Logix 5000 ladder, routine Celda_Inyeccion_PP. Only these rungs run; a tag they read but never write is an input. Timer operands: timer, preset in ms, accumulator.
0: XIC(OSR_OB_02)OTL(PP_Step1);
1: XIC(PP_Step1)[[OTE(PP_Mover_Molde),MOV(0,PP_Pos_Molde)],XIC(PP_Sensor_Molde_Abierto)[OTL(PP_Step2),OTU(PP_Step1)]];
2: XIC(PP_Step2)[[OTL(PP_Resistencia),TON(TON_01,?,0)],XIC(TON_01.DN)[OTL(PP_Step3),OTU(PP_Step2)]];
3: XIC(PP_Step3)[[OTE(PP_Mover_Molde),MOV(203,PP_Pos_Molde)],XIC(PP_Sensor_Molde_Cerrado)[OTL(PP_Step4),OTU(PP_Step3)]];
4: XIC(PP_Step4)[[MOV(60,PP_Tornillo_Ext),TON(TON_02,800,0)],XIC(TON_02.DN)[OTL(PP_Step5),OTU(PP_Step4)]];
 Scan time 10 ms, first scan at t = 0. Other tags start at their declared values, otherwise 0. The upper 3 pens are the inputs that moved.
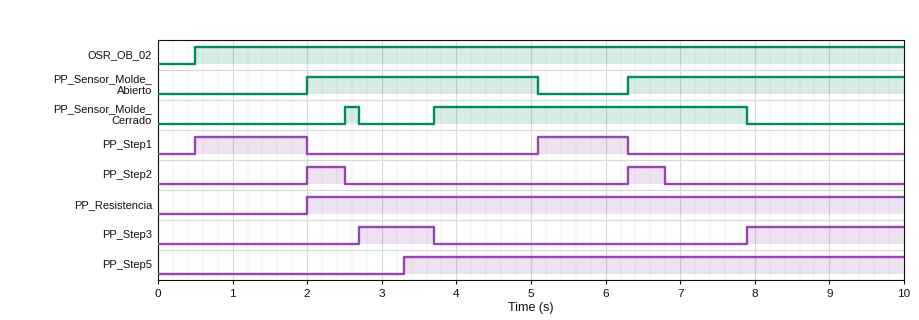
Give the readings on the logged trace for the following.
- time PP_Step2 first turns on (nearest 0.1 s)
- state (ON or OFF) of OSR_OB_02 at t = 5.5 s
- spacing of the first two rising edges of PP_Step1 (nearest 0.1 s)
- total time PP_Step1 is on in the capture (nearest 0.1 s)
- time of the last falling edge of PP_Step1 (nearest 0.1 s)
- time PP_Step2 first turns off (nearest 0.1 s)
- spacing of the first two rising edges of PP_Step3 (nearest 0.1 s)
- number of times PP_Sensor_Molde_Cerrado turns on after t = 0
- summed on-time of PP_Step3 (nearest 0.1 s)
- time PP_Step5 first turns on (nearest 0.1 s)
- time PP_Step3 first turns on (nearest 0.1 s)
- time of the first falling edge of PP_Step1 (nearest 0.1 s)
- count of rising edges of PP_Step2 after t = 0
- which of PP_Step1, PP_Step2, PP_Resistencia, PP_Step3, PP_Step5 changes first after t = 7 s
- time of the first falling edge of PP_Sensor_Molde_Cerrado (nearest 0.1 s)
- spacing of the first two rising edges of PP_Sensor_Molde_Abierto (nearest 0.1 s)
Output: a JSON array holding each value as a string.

["2.0 s", "ON", "4.6 s", "2.7 s", "6.3 s", "2.5 s", "5.2 s", "2", "3.1 s", "3.3 s", "2.7 s", "2.0 s", "2", "PP_Step3", "2.7 s", "4.3 s"]
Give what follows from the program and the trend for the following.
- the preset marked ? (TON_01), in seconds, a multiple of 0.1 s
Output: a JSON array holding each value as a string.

["0.5 s"]
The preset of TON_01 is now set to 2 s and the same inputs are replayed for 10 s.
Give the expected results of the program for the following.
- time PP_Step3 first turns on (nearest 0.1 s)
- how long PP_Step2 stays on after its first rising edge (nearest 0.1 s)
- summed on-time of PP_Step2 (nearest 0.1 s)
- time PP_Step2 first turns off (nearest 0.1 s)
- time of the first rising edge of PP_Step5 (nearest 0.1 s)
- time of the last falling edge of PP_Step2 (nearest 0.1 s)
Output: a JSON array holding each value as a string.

["8.3 s", "2.0 s", "4.0 s", "4.0 s", "4.8 s", "8.3 s"]
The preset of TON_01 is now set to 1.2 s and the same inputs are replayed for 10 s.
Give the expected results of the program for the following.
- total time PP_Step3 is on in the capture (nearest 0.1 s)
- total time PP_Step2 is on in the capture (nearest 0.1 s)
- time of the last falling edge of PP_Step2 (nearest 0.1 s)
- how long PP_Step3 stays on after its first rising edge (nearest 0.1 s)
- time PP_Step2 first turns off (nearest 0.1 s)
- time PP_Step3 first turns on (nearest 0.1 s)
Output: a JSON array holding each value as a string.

["2.6 s", "2.4 s", "7.5 s", "0.5 s", "3.2 s", "3.2 s"]
